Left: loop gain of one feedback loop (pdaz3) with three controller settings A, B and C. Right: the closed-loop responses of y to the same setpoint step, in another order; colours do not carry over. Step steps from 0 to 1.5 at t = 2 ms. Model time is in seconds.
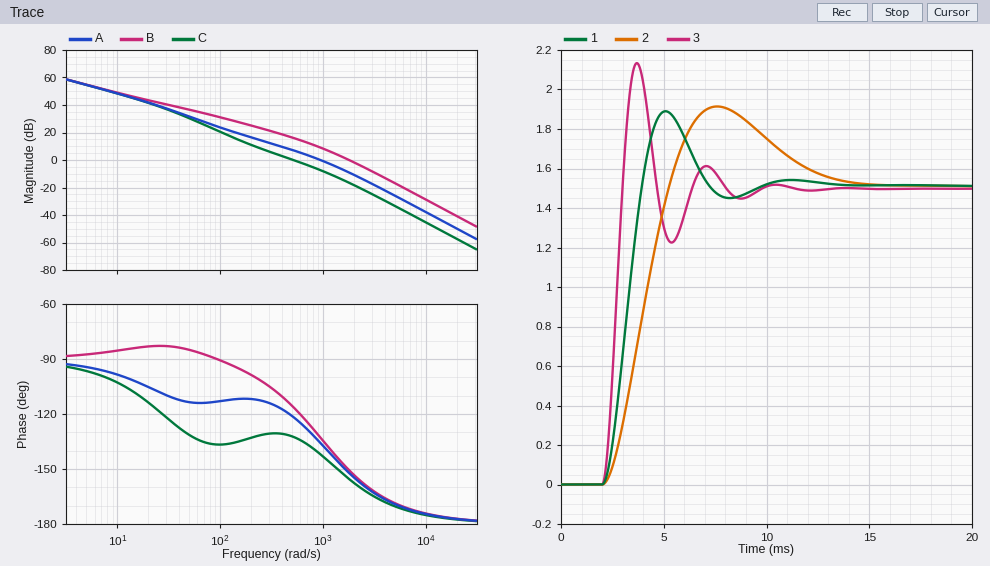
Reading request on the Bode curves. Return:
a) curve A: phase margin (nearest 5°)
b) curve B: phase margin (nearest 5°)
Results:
45°
30°
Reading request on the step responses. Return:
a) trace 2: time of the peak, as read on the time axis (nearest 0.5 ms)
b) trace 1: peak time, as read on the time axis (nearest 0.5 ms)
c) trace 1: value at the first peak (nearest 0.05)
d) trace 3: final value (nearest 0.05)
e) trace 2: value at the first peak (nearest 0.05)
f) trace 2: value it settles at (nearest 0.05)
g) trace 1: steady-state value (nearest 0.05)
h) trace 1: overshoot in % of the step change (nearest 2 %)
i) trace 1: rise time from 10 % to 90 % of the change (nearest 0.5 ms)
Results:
7.5 ms
5.0 ms
1.90
1.50
1.90
1.50
1.50
26 %
1.5 ms
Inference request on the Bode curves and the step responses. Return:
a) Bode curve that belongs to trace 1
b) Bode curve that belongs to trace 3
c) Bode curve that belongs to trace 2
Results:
A
B
C
